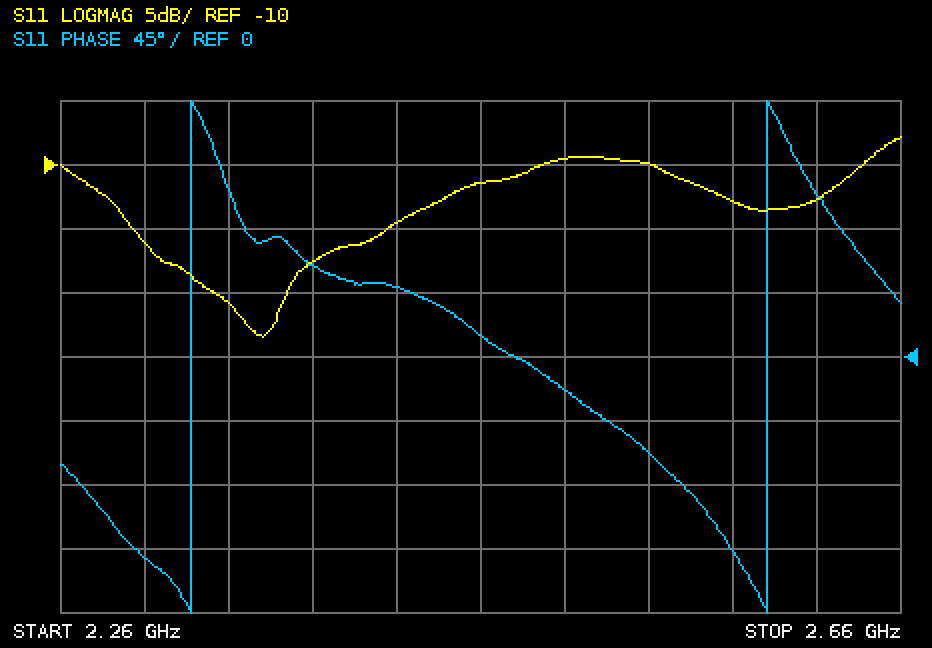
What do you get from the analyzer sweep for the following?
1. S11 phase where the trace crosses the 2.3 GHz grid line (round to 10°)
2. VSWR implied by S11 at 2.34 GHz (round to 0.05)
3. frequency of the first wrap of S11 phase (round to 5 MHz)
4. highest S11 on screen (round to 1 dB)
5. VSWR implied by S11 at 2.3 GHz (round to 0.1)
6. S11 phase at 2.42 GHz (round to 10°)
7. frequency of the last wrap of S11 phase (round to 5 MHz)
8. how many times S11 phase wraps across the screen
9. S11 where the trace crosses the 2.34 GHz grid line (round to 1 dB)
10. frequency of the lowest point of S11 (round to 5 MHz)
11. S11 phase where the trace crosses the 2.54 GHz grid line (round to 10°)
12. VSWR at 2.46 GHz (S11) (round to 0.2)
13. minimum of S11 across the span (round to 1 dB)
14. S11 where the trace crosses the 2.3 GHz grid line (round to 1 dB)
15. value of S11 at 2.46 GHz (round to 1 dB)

-140°
1.20
2.320 GHz
-8 dB
1.4
50°
2.595 GHz
2
-21 dB
2.355 GHz
-70°
1.8
-23 dB
-16 dB
-11 dB
